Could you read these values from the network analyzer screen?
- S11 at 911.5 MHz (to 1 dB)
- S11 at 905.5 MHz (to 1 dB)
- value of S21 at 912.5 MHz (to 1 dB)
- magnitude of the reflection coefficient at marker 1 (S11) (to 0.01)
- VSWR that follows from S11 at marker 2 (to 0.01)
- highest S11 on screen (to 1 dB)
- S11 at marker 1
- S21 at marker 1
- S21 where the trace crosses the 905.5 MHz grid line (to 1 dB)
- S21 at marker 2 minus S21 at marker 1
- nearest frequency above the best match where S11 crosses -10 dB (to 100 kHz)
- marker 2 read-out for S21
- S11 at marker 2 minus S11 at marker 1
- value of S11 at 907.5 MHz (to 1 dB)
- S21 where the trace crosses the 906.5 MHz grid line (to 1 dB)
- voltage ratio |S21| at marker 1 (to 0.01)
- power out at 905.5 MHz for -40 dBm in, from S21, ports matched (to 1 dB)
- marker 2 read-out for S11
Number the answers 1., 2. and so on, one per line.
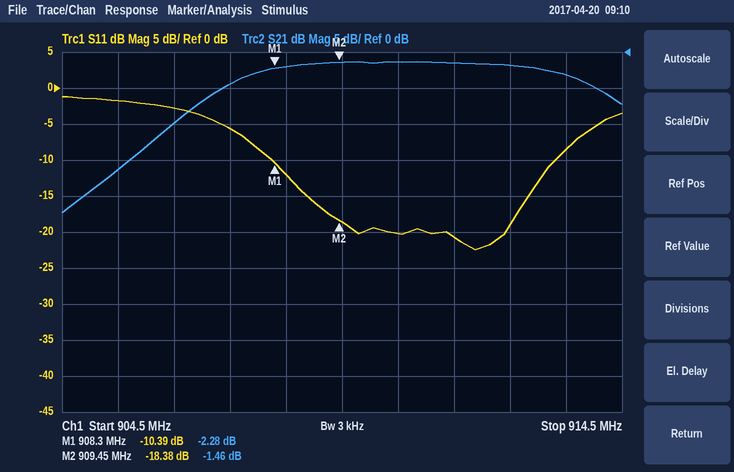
1. -21 dB
2. -2 dB
3. -2 dB
4. 0.30
5. 1.27
6. -1 dB
7. -10.39 dB
8. -2.28 dB
9. -16 dB
10. 0.82 dB
11. 913.3 MHz
12. -1.46 dB
13. -7.99 dB
14. -6 dB
15. -10 dB
16. 0.77
17. -56 dBm
18. -18.38 dB
